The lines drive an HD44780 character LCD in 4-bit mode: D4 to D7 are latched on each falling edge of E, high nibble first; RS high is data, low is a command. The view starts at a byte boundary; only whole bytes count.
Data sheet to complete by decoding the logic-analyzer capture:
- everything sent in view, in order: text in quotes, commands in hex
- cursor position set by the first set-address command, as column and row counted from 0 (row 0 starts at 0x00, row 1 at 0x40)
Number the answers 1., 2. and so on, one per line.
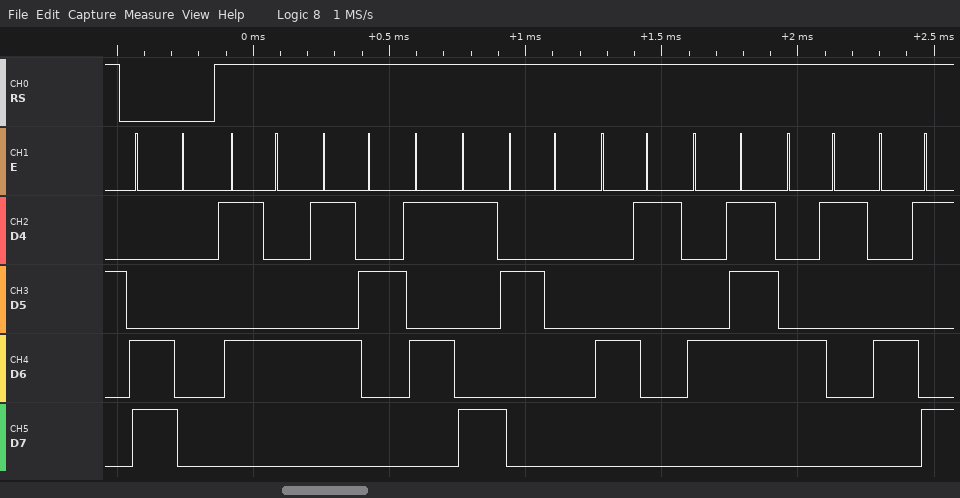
1. 0xC0 "TRY AGAI"
2. column 0, row 1
